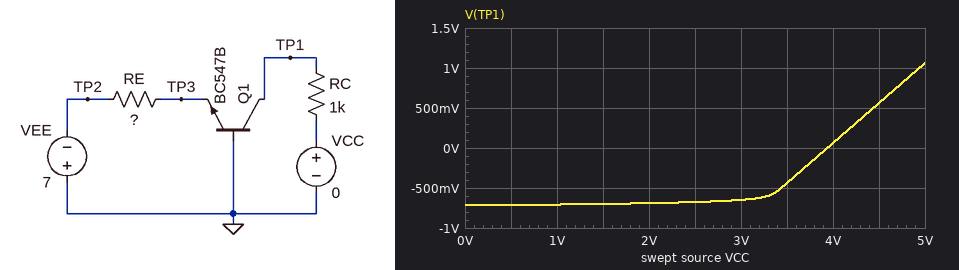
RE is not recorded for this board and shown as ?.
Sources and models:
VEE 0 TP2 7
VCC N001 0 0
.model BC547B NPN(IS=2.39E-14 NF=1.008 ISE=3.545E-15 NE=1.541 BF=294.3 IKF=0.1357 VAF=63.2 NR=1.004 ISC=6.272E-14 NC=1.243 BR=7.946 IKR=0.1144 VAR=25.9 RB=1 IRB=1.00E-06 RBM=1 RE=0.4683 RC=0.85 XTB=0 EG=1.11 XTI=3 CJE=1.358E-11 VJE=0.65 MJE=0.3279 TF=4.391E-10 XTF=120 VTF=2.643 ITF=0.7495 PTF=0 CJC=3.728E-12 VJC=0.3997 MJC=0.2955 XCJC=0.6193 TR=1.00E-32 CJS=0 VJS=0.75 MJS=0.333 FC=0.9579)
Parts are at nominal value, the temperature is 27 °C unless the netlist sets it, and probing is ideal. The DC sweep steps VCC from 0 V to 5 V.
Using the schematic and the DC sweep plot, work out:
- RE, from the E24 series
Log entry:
1.6 kΩ
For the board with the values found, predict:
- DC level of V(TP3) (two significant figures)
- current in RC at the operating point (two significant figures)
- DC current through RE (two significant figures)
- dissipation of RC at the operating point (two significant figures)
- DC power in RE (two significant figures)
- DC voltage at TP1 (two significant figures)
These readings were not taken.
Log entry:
-730 mV
720 µA
3.9 mA
520 µW
25 mW
-720 mV
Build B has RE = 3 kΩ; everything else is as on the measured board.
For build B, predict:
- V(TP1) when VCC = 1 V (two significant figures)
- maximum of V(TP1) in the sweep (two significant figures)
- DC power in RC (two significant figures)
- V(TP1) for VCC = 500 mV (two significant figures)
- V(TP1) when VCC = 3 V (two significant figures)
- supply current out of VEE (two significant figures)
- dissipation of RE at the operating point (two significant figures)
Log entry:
-660 mV
2.9 V
480 µW
-680 mV
890 mV
2.1 mA
13 mW
